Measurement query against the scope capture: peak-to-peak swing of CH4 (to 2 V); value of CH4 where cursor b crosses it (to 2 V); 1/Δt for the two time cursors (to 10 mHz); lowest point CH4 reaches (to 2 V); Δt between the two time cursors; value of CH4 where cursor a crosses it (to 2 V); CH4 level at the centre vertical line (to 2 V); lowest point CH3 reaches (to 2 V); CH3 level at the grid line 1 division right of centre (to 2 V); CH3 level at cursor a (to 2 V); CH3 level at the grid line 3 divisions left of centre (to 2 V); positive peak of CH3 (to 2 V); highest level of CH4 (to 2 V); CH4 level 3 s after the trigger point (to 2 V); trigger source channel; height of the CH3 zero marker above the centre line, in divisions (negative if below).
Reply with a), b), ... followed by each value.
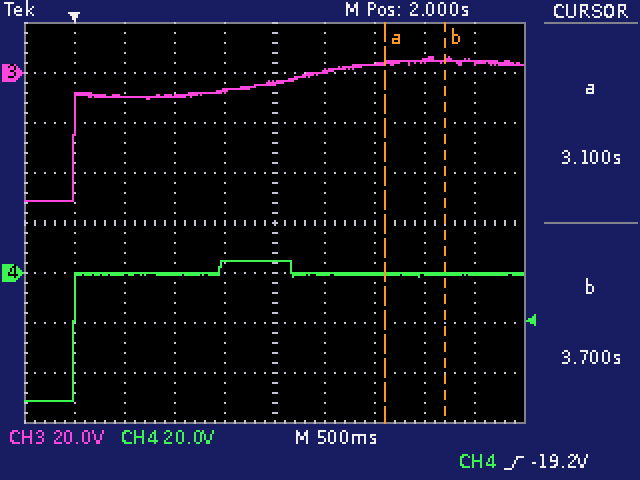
a) 56 V
b) 0 V
c) 1.67 Hz
d) -52 V
e) 600 ms
f) 0 V
g) 4 V
h) -52 V
i) 0 V
j) 4 V
k) -10 V
l) 6 V
m) 4 V
n) 0 V
o) CH4
p) +3.0 div
